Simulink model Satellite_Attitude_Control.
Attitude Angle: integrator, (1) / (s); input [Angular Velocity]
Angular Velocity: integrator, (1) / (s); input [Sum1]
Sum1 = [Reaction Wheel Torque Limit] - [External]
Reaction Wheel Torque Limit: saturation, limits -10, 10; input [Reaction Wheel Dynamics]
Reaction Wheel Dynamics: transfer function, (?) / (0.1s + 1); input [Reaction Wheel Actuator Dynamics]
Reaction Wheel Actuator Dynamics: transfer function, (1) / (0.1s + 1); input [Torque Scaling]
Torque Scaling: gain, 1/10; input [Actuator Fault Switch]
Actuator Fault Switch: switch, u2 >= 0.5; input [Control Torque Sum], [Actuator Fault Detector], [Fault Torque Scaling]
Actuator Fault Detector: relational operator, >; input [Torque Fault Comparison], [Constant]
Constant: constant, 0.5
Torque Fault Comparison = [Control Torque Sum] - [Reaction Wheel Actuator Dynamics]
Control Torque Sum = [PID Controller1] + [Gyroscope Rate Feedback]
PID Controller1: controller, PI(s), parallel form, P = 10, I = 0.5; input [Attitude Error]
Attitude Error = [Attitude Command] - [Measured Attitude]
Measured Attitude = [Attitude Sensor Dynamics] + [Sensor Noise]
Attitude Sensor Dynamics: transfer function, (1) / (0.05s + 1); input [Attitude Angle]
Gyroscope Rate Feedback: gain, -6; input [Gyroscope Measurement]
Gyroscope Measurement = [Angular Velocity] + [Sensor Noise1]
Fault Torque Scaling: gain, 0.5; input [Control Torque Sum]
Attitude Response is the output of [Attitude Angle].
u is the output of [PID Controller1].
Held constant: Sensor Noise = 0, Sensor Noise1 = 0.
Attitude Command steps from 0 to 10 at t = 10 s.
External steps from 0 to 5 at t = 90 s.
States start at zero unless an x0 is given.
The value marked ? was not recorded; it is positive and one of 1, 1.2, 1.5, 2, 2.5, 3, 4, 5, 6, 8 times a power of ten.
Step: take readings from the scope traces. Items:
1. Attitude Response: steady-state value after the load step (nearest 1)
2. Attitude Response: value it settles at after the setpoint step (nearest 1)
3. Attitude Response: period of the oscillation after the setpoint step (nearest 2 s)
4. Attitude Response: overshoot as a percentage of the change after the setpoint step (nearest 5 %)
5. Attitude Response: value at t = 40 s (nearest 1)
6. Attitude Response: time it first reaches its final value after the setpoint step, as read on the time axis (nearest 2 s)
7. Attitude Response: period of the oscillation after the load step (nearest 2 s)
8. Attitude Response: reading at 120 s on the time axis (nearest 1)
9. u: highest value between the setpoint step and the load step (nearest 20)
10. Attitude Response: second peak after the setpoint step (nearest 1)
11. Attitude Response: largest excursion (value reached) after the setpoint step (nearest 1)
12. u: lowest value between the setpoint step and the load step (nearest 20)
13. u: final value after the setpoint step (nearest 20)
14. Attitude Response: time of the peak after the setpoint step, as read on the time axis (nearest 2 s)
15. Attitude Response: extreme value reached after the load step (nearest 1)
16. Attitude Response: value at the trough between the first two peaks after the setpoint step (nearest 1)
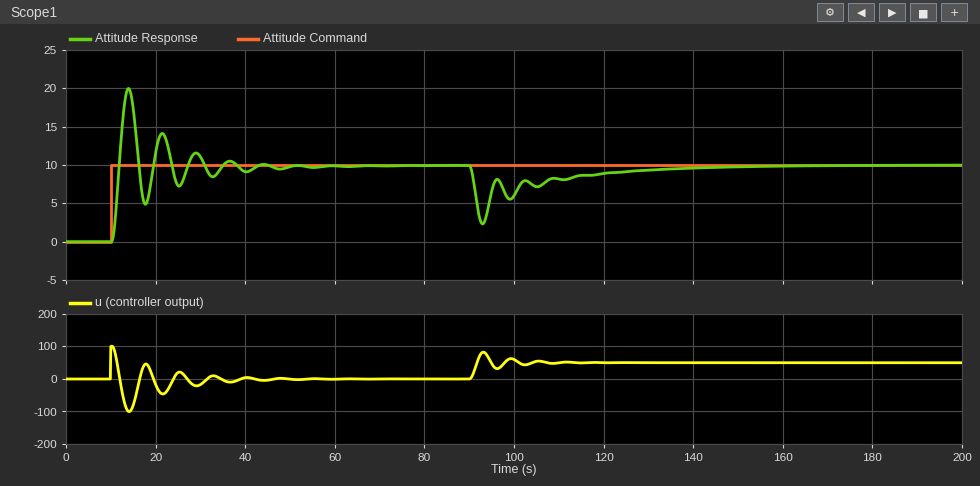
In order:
10
10
8 s
100 %
9
12 s
6 s
9
100
14
20
-100
0
14 s
2
5
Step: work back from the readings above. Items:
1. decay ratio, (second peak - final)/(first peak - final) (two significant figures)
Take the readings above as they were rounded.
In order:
0.40
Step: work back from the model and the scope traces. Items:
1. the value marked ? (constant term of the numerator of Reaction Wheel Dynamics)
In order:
1
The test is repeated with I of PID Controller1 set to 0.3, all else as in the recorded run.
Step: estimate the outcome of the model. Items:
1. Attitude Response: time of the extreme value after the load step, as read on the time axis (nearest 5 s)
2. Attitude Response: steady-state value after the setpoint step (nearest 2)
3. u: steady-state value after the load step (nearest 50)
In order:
95 s
10
50
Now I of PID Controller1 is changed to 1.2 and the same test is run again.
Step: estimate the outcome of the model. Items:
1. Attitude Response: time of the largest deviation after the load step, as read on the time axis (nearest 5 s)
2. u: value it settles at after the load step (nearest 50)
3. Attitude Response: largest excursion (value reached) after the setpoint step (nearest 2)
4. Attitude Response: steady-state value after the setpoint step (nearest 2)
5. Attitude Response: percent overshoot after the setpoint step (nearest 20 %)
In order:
95 s
50
22
10
120 %
